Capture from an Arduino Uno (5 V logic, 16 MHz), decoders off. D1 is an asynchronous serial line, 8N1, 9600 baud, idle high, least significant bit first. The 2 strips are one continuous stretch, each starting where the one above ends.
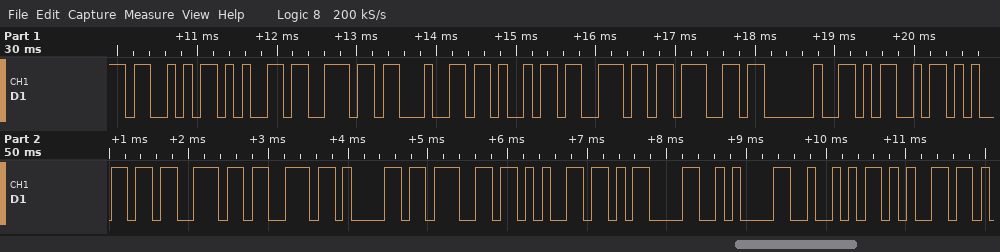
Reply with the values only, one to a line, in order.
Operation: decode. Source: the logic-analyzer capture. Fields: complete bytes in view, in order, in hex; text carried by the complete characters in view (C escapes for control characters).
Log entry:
53 65 6E 64 69 6E 67 20 4D 65 73 73 61 67 65 0D 0A 52 65
"Sending Message\r\nRe"
